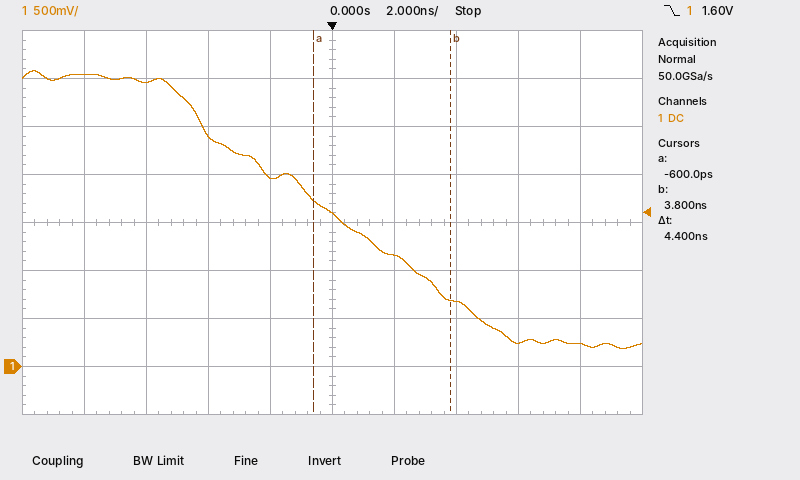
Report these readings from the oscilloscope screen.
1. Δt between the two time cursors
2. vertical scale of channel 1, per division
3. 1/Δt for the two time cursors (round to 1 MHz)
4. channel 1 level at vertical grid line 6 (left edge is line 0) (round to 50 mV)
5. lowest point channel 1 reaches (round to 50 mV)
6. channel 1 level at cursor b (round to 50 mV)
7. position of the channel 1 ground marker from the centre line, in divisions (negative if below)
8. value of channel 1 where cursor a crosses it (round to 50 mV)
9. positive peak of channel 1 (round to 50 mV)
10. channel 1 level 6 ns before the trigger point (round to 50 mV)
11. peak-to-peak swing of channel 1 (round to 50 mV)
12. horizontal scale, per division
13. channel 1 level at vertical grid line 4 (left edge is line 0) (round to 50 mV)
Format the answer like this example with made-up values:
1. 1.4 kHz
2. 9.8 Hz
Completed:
1. 4.4 ns
2. 500 mV
3. 227 MHz
4. 1.15 V
5. 200 mV
6. 700 mV
7. -3.0 div
8. 1.75 V
9. 3.10 V
10. 2.95 V
11. 2.90 V
12. 2 ns
13. 1.95 V
